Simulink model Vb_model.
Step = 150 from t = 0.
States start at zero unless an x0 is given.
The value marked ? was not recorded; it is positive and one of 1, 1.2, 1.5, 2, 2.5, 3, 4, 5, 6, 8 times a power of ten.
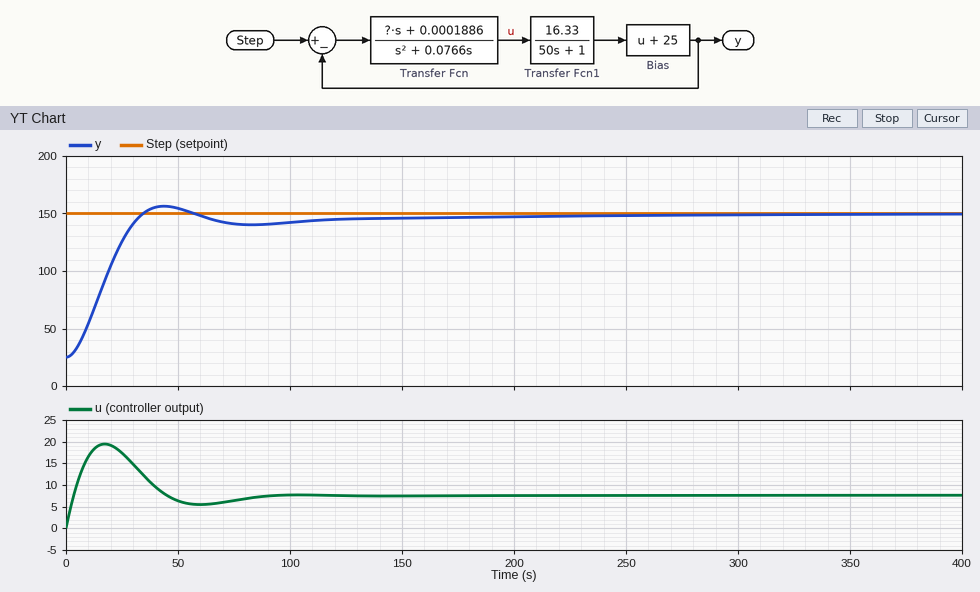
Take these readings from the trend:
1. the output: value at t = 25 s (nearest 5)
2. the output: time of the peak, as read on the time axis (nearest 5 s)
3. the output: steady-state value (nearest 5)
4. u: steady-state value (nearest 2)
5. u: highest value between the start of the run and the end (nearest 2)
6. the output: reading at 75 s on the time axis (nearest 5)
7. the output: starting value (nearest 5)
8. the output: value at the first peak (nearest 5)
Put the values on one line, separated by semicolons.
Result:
125; 45 s; 150; 8; 20; 140; 25; 155
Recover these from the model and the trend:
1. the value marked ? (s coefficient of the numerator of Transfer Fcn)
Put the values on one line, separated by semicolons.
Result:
0.02
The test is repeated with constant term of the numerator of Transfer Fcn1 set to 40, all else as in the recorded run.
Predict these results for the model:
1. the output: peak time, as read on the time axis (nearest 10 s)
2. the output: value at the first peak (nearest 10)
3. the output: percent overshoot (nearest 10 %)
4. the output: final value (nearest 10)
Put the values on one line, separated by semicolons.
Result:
30 s; 180; 30 %; 150
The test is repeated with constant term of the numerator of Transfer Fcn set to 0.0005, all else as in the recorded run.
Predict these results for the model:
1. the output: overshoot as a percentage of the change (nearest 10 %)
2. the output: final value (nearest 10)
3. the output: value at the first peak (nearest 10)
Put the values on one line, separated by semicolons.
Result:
20 %; 150; 180
